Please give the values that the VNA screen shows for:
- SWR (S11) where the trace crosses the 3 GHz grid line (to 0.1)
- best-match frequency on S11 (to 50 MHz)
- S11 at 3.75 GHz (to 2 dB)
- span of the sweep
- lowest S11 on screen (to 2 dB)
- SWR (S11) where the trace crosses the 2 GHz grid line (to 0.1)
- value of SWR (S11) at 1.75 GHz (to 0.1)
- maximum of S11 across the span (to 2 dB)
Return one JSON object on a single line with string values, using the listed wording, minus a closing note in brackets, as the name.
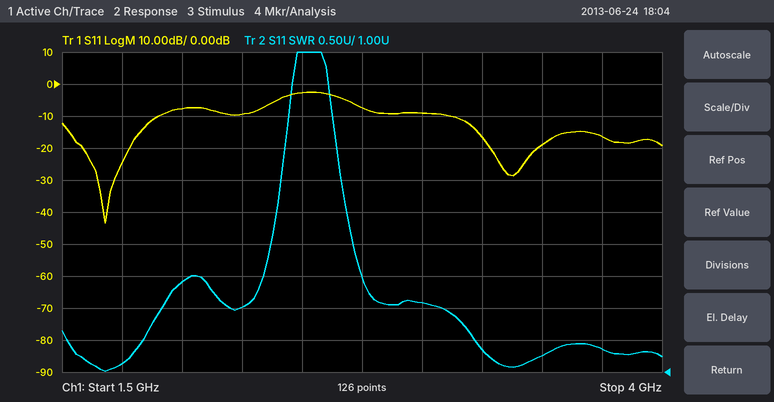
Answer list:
{"SWR (S11) where the trace crosses the 3 GHz grid line": "2.1", "best-match frequency on S11": "1.70 GHz", "S11 at 3.75 GHz": "-16 dB", "span of the sweep": "2.5 GHz", "lowest S11 on screen": "-44 dB", "SWR (S11) where the trace crosses the 2 GHz grid line": "2.4", "value of SWR (S11) at 1.75 GHz": "1.1", "maximum of S11 across the span": "-2 dB"}
